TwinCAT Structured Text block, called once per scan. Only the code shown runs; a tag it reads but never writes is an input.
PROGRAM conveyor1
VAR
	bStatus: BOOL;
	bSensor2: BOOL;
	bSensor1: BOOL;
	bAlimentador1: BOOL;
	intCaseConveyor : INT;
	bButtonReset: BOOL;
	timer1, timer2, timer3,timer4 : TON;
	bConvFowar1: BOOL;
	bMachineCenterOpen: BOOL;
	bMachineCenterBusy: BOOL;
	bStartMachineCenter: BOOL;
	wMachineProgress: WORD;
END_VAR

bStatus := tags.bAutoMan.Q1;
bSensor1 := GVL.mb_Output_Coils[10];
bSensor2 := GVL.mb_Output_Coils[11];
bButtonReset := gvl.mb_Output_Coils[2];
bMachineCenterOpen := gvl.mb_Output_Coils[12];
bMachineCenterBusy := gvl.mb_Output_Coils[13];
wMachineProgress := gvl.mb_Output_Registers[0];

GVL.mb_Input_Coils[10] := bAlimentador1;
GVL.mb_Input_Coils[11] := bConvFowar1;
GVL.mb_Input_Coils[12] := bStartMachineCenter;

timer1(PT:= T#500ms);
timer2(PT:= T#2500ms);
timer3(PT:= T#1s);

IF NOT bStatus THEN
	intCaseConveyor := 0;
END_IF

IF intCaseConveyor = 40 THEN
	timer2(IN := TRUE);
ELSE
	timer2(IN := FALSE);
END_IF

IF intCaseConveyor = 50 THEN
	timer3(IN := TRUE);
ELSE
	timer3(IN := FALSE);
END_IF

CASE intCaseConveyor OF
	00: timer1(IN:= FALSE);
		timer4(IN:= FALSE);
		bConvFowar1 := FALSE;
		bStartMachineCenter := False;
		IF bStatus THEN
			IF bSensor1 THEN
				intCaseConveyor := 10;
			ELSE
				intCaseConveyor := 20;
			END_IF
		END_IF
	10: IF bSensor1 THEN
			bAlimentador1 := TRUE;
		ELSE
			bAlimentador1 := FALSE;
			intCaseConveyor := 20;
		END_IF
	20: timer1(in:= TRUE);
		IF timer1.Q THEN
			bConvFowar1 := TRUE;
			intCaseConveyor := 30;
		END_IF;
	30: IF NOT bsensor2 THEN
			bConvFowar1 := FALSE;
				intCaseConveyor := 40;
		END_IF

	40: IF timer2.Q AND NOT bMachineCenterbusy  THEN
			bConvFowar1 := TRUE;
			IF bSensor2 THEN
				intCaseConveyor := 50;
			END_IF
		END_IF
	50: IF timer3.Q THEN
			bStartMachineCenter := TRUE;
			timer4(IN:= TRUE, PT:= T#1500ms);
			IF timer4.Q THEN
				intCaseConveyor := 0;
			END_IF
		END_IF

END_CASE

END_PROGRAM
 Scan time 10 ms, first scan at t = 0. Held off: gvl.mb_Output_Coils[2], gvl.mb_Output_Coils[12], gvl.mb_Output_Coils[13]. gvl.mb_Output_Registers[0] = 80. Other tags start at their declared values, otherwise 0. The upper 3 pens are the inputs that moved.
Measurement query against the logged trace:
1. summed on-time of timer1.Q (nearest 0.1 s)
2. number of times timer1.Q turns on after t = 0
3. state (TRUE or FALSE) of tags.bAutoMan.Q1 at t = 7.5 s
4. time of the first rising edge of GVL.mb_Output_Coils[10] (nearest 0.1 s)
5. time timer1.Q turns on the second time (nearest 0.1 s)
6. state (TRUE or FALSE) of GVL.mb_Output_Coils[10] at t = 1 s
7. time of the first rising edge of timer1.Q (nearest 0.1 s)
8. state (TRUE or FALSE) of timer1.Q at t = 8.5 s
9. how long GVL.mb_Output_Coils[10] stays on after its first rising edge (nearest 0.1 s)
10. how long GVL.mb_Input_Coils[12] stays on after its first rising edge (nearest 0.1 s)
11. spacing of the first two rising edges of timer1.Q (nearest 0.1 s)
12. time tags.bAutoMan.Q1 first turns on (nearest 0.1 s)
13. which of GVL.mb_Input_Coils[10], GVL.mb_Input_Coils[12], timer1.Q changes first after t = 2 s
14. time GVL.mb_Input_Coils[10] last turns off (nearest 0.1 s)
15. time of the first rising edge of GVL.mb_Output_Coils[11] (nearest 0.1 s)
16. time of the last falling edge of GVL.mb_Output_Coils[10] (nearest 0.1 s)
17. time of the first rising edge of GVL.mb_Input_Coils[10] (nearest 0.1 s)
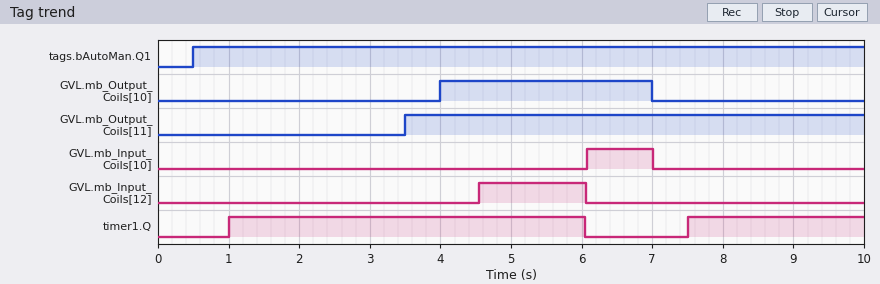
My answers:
7.5 s
2
TRUE
4.0 s
7.5 s
FALSE
1.0 s
TRUE
3.0 s
1.5 s
6.5 s
0.5 s
GVL.mb_Input_Coils[12]
7.0 s
3.5 s
7.0 s
6.1 s
